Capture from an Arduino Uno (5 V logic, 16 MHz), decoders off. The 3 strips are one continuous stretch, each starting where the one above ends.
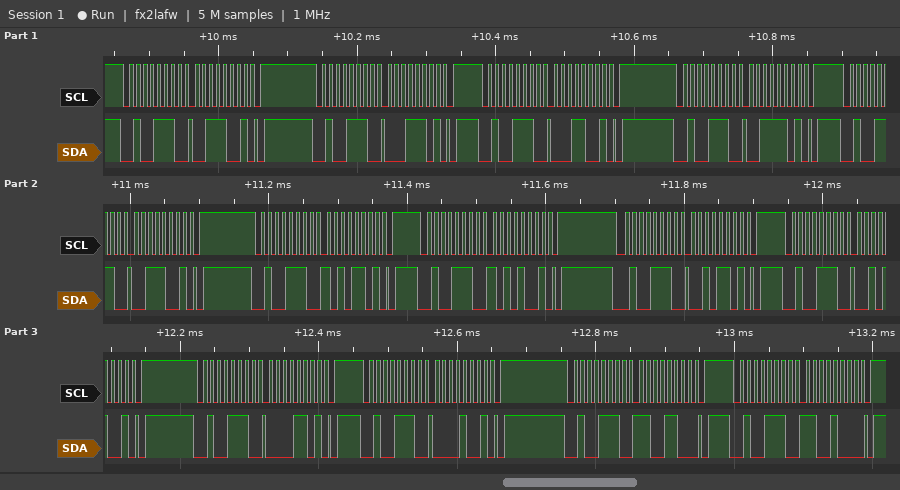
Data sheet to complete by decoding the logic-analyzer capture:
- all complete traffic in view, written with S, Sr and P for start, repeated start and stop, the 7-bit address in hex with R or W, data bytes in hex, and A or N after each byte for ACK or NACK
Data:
S 27W A 39 A P S 27W A 1D A P S 27W A 19 A P S 27W A 3D A P S 27W A 39 A P S 27W A AD A P S 27W A A9 A P S 27W A 2D A P S 27W A 29 A P S 27W A 0D A P S 27W A 09 A P S 27W A CC A P S 27W A C8 A P
